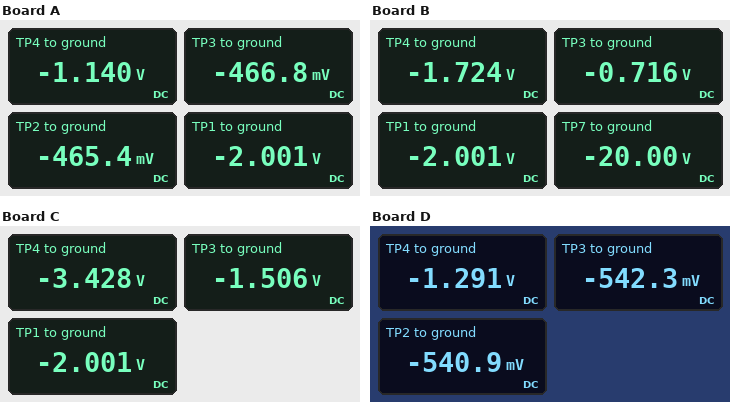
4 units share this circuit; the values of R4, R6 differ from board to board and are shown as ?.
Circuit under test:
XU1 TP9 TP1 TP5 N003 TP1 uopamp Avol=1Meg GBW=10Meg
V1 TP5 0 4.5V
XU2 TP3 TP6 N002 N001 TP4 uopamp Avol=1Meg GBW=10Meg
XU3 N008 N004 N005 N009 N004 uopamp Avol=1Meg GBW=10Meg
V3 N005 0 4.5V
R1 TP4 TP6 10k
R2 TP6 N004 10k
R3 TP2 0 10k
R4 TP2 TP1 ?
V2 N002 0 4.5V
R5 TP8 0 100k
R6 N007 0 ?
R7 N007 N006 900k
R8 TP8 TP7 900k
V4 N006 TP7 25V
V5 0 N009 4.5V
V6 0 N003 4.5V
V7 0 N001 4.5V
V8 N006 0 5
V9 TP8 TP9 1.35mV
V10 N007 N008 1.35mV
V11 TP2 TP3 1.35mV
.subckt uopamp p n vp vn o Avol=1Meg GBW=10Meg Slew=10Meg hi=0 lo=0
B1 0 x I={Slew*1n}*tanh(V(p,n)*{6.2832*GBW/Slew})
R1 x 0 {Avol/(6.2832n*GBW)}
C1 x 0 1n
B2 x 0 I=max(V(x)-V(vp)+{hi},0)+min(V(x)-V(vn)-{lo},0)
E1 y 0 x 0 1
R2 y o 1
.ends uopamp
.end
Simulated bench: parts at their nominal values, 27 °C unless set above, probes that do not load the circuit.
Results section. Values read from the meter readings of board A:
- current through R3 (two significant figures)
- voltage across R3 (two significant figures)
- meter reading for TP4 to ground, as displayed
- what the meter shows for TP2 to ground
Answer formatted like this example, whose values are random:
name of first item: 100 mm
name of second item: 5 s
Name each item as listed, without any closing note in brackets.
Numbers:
current through R3: 47 µA
voltage across R3: 470 mV
meter reading for TP4 to ground, as displayed: -1.140 V
what the meter shows for TP2 to ground: -465.4 mV
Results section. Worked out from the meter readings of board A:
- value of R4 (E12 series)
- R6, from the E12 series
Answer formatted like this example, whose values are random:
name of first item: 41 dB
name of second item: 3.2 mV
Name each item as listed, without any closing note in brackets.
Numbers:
value of R4: 33 kΩ
R6, from the E12 series: 39 kΩ
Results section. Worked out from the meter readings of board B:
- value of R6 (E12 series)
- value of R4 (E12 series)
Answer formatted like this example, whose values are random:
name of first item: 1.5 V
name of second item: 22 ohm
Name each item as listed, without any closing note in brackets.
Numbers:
value of R6: 56 kΩ
value of R4: 18 kΩ
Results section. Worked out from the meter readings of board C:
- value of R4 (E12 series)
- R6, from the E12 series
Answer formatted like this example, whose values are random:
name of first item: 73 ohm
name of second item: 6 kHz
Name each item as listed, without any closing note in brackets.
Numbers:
value of R4: 3.3 kΩ
R6, from the E12 series: 82 kΩ
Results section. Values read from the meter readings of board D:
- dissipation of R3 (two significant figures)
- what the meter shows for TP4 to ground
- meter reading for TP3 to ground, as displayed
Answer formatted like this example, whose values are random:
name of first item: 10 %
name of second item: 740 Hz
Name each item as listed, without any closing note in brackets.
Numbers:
dissipation of R3: 29 µW
what the meter shows for TP4 to ground: -1.291 V
meter reading for TP3 to ground, as displayed: -542.3 mV
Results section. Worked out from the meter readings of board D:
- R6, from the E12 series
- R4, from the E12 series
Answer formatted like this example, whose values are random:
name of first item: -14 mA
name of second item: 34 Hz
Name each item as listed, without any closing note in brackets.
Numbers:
R6, from the E12 series: 39 kΩ
R4, from the E12 series: 27 kΩ
